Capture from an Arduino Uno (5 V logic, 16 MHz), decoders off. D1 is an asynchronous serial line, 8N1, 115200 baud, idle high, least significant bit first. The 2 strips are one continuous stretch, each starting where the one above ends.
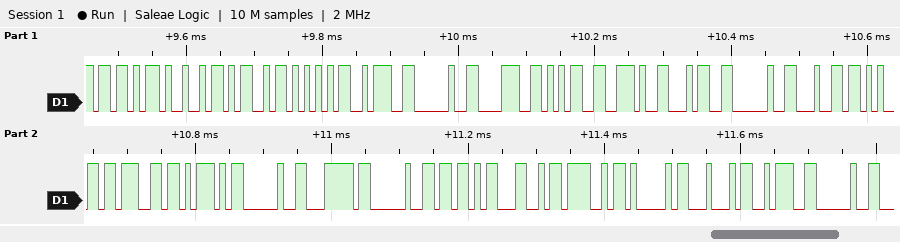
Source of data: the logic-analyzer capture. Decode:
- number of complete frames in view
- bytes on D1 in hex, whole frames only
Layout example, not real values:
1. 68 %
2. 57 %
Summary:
1. 25
2. 5B 49 4D 55 3A 20 38 35 2E 34 20 64 65 67 5D 20 7C 20 5B 4C 4F 41 44 3A 20
